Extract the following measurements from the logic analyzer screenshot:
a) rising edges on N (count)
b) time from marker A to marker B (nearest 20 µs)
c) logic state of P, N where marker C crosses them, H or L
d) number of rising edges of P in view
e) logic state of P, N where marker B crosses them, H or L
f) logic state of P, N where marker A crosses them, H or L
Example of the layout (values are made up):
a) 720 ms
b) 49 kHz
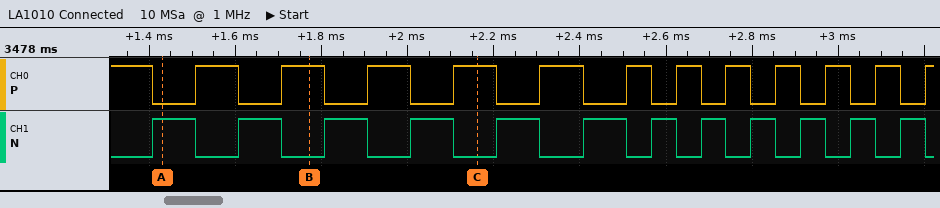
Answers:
a) 12
b) 340 µs
c) P=H, N=L
d) 12
e) P=H, N=L
f) P=L, N=H
